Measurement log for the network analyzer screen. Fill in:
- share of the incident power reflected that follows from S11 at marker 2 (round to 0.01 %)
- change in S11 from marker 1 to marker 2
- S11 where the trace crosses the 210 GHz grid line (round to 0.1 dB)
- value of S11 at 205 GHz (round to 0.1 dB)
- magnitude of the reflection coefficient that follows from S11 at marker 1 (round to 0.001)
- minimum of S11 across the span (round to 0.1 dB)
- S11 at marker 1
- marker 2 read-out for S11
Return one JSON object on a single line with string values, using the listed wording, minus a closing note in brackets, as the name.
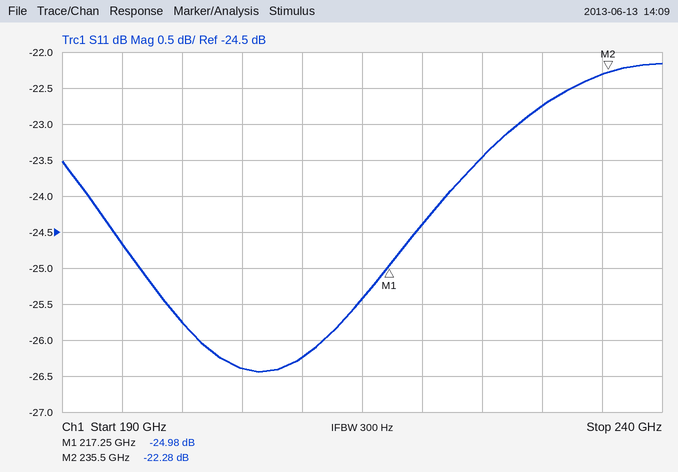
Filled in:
{"share of the incident power reflected that follows from S11 at marker 2": "0.59 %", "change in S11 from marker 1 to marker 2": "2.70 dB", "S11 where the trace crosses the 210 GHz grid line": "-26.2 dB", "value of S11 at 205 GHz": "-26.4 dB", "magnitude of the reflection coefficient that follows from S11 at marker 1": "0.056", "minimum of S11 across the span": "-26.4 dB", "S11 at marker 1": "-24.98 dB", "marker 2 read-out for S11": "-22.28 dB"}
